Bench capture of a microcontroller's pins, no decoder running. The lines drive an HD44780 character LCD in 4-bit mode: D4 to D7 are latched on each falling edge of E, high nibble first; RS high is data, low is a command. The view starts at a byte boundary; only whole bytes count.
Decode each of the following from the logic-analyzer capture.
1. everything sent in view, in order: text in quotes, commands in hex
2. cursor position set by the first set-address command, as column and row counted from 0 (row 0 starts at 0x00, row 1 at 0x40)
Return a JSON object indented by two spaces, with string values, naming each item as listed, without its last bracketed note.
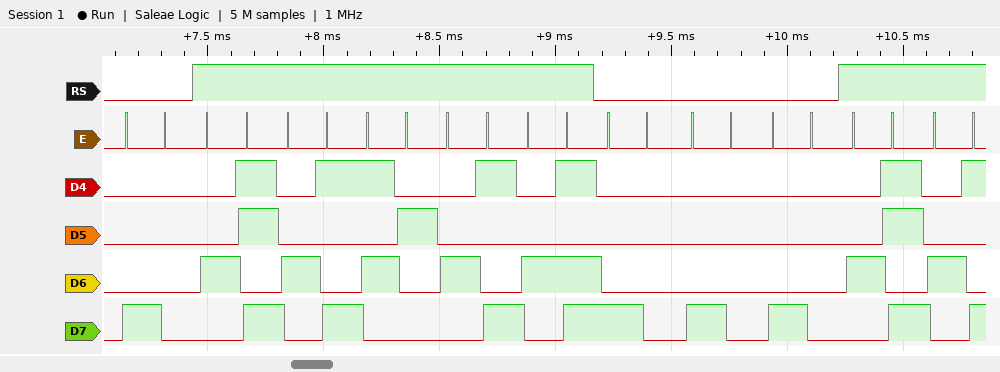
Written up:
{
  "everything sent in view, in order: text in quotes, commands in hex": "0x80 \"KIRIM\" 0x80 0x80 0x80 \"KI\"",
  "cursor position set by the first set-address command, as column and row counted from 0": "column 0, row 0"
}
